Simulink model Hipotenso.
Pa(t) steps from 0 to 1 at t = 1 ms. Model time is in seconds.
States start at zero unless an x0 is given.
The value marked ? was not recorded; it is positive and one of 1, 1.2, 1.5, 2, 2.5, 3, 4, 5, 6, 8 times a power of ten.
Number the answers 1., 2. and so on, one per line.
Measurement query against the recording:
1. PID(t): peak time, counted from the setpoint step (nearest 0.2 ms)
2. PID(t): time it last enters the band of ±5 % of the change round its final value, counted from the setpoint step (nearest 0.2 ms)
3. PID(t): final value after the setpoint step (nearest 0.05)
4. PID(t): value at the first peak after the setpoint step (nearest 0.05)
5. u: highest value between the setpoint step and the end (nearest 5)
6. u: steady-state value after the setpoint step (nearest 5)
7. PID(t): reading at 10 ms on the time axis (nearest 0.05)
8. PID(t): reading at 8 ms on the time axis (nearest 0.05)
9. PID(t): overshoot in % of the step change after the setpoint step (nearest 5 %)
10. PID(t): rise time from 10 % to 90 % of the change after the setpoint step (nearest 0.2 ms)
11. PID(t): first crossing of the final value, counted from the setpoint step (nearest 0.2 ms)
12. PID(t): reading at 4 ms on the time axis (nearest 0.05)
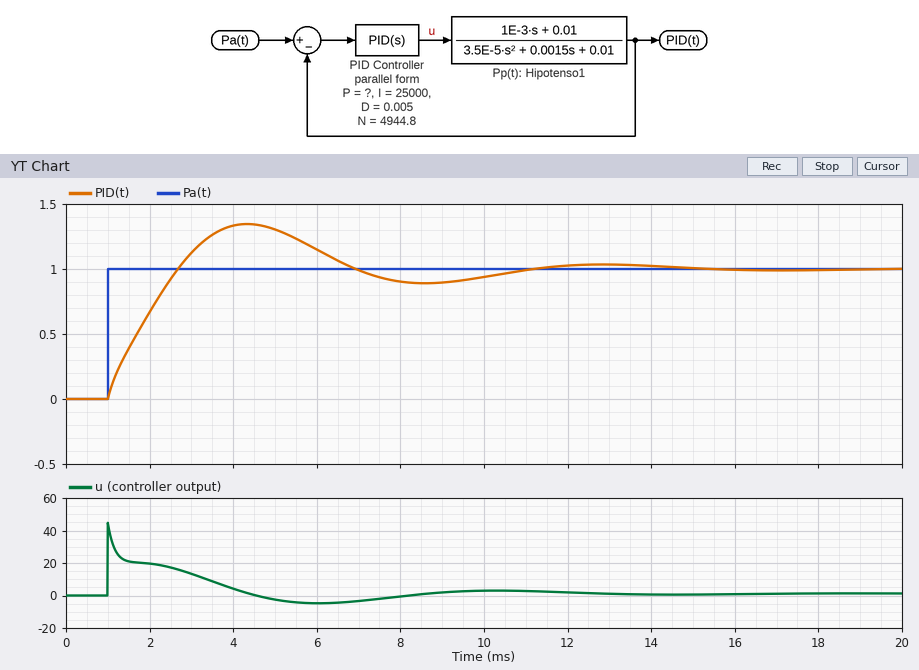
1. 3.4 ms
2. 9.2 ms
3. 1.00
4. 1.35
5. 45
6. 0
7. 0.95
8. 0.90
9. 35 %
10. 1.4 ms
11. 1.6 ms
12. 1.35
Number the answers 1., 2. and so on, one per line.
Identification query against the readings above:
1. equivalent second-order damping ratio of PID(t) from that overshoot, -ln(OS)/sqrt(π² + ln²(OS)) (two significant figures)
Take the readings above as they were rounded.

1. 0.32
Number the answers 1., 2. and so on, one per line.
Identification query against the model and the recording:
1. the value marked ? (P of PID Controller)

1. 20
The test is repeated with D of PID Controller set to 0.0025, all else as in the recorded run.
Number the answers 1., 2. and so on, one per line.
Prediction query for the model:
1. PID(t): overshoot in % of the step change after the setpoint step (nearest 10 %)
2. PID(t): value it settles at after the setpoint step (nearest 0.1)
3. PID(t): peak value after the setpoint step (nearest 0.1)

1. 40 %
2. 1.0
3. 1.4
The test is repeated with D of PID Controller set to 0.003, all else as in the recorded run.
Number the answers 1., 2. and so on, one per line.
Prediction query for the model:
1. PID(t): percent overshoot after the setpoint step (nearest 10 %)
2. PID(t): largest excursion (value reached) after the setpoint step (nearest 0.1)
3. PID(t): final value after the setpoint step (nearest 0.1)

1. 40 %
2. 1.4
3. 1.0
